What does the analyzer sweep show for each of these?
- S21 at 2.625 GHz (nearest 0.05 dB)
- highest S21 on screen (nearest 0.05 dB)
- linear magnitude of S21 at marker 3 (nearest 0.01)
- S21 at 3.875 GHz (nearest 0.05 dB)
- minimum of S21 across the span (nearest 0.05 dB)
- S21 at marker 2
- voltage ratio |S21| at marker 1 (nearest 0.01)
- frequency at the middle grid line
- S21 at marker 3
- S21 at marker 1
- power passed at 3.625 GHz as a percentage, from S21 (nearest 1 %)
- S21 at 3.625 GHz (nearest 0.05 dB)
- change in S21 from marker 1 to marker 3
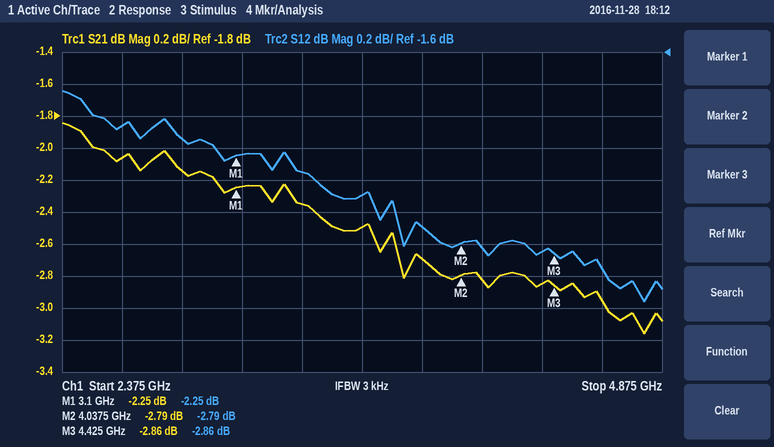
-2.05 dB
-1.85 dB
0.72
-2.70 dB
-3.15 dB
-2.79 dB
0.77
3.625 GHz
-2.86 dB
-2.25 dB
56 %
-2.50 dB
-0.61 dB
